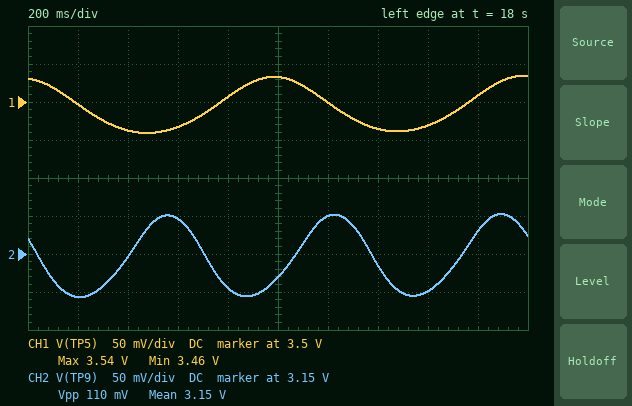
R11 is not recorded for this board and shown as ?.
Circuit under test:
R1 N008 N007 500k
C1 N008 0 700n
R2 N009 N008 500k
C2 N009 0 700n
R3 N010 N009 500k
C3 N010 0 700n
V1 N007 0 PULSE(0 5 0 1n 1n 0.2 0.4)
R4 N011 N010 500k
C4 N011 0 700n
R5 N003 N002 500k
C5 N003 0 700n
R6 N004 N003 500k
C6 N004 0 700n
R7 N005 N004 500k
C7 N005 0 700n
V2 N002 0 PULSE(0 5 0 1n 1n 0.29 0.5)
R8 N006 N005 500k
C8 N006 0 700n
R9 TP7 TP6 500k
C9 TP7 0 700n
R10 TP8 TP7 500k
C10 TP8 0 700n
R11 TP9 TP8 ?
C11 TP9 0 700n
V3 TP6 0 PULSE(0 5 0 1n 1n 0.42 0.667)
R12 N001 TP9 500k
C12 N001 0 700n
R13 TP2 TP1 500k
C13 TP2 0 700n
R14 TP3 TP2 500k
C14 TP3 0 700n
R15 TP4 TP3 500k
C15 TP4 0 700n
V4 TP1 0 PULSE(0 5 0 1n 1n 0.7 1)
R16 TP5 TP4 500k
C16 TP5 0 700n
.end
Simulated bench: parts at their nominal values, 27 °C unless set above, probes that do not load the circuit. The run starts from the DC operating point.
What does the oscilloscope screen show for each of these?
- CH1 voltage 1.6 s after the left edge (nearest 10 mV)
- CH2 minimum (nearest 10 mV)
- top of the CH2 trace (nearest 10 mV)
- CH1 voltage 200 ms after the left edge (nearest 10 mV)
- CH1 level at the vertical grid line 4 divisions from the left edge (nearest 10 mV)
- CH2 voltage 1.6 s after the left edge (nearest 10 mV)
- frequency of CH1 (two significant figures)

3.47 V
3.09 V
3.20 V
3.50 V
3.51 V
3.10 V
1.0 Hz
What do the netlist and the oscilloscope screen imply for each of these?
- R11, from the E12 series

390 kΩ
